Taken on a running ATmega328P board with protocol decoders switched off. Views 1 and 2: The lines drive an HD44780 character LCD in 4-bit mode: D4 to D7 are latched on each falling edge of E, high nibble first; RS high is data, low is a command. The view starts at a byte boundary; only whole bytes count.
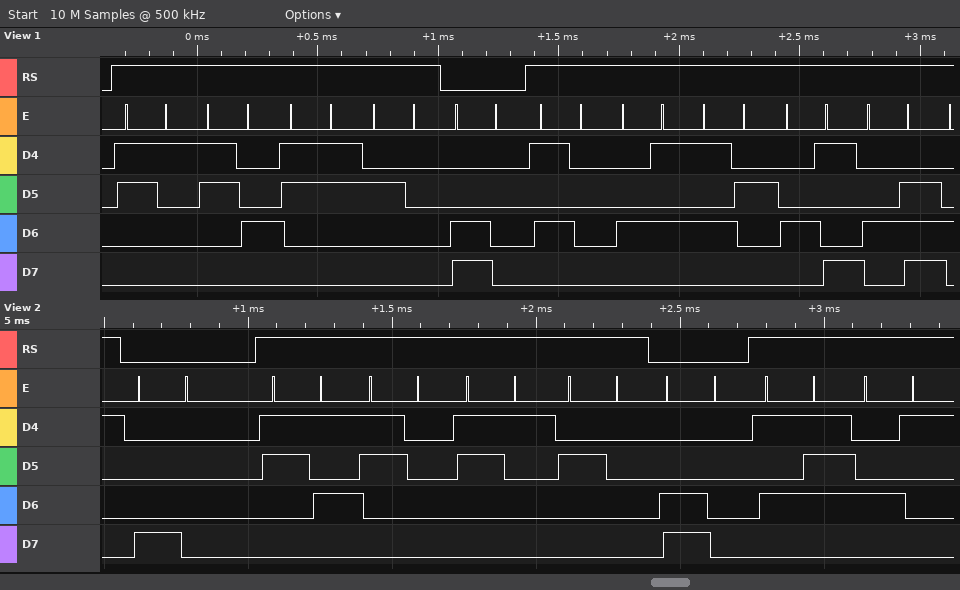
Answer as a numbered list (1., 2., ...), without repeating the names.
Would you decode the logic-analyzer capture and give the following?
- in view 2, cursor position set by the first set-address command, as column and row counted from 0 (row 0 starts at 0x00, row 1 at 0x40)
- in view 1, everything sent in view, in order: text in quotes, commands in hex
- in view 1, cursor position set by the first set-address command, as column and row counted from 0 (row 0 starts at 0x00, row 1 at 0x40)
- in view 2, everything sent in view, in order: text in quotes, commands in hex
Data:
1. column 0, row 0
2. "143 " 0xC0 "PERIN"
3. column 0, row 1
4. 0x80 "501 " 0xC0 "WA"
